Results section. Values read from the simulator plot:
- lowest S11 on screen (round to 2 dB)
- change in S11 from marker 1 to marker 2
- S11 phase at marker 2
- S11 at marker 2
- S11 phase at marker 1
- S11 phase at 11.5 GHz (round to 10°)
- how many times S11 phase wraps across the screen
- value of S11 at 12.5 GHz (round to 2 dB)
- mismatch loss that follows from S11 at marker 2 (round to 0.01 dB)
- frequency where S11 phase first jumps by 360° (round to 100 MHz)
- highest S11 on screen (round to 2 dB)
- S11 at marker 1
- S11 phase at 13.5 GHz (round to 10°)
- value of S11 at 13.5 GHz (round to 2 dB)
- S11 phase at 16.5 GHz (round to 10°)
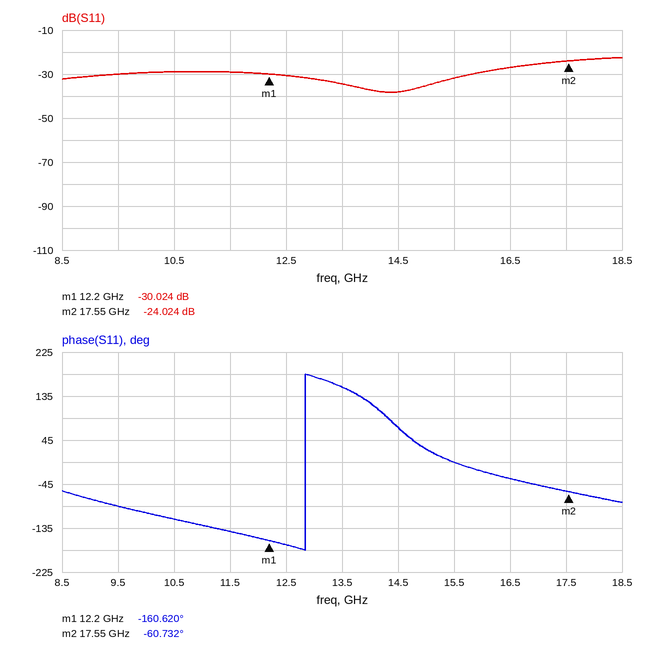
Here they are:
-38 dB
6.000 dB
-60.732°
-24.024 dB
-160.620°
-140°
1
-30 dB
0.02 dB
12.8 GHz
-22 dB
-30.024 dB
150°
-34 dB
-30°
